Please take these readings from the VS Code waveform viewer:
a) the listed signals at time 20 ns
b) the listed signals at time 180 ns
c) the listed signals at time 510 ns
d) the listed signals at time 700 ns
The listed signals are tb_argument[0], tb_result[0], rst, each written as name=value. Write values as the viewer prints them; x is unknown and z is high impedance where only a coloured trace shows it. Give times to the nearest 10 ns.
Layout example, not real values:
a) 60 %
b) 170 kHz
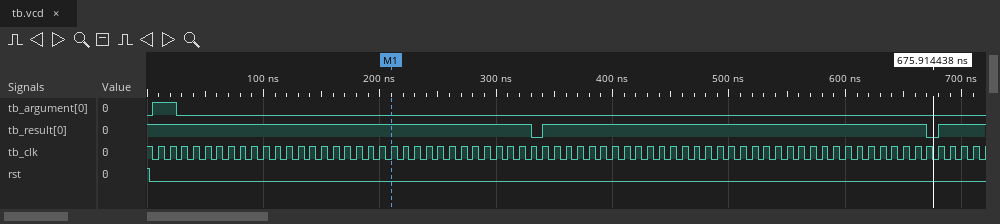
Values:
a) tb_argument[0]=1, tb_result[0]=1, rst=0
b) tb_argument[0]=0, tb_result[0]=1, rst=0
c) tb_argument[0]=0, tb_result[0]=1, rst=0
d) tb_argument[0]=0, tb_result[0]=1, rst=0
